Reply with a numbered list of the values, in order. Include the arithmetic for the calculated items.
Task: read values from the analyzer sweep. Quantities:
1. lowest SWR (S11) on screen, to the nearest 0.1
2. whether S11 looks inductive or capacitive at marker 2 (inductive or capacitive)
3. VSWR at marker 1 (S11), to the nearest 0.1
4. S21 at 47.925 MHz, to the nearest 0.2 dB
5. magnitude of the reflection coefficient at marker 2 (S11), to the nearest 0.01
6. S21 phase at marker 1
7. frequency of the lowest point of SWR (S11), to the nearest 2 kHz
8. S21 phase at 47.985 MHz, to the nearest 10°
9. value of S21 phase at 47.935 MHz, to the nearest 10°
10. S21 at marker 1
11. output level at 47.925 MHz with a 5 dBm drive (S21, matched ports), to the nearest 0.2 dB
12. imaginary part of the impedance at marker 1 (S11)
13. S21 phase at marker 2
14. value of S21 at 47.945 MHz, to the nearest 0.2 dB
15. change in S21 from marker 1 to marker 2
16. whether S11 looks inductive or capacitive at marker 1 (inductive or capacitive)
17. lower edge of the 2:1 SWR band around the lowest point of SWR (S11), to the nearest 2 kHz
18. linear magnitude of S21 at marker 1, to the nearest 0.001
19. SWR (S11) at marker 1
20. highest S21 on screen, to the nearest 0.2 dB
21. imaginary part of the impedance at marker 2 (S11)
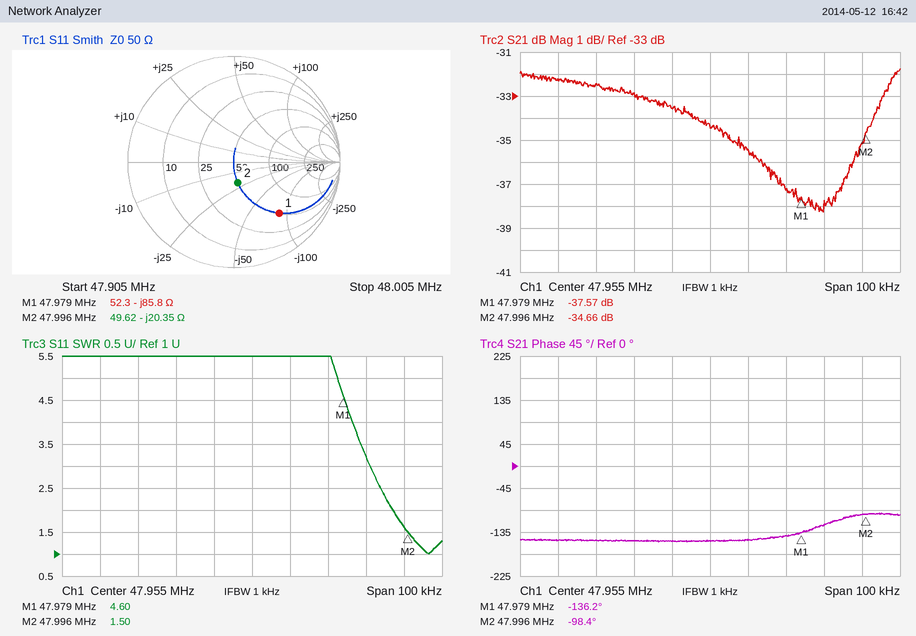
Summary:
1. 1.0
2. capacitive
3. 4.6
4. -32.4 dB
5. 0.20
6. -136.2°
7. 48.002 MHz
8. -120°
9. -150°
10. -37.57 dB
11. 5 dBm + (-32.4 dB) = -27.4 dBm
12. -85.8 Ω
13. -98.4°
14. -33.6 dB
15. -34.66 − (-37.57) = 2.91 dB
16. capacitive
17. 47.992 MHz
18. 10^(-37.57/20) ≈ 0.013
19. 4.60
20. -31.8 dB
21. -20.35 Ω
